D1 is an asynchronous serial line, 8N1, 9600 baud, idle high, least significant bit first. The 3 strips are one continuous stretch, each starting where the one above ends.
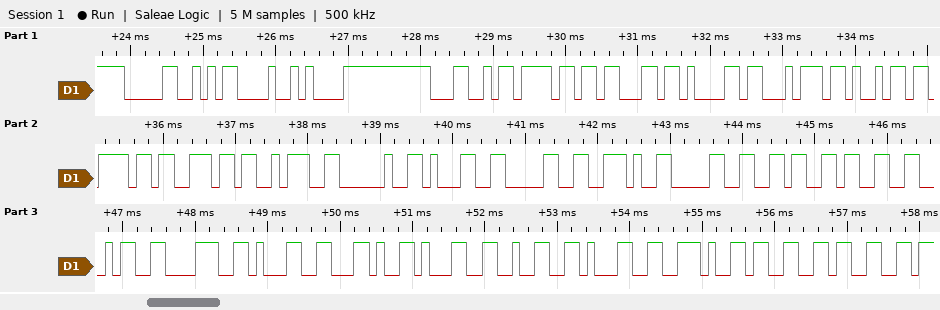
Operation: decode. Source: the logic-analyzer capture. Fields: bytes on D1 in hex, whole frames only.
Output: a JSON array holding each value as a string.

["30 0D 0A 4C 6F 63 61 74 69 6F 6E 3A 20 31 30 2E 30 36 33 34 38 31 2C 31 32 31 2E 33 33"]
